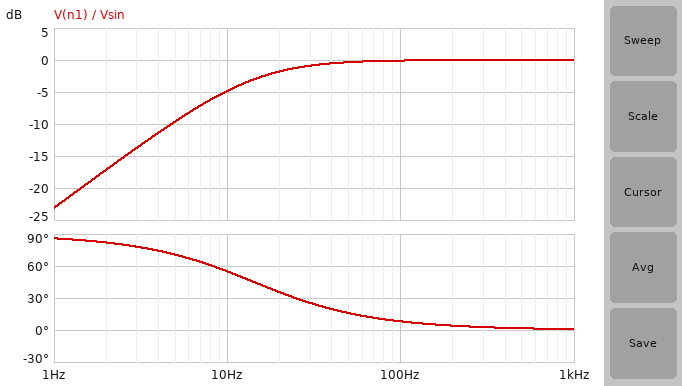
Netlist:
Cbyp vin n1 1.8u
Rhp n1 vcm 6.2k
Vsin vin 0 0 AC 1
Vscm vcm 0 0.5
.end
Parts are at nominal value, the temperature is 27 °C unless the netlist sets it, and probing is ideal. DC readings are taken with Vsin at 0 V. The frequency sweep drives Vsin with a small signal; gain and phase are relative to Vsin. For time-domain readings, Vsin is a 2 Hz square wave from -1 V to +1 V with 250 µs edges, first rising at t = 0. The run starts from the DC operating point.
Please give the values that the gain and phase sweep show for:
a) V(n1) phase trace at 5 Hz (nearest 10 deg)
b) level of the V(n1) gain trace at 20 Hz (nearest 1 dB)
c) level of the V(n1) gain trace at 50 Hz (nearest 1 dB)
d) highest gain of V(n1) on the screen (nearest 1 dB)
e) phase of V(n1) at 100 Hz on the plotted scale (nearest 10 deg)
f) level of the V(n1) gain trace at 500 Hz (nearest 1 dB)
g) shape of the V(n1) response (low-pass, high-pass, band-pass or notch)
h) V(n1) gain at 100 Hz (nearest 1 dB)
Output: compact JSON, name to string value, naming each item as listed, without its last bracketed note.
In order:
{"V(n1) phase trace at 5 Hz": "70 deg", "level of the V(n1) gain trace at 20 Hz": "-2 dB", "level of the V(n1) gain trace at 50 Hz": "0 dB", "highest gain of V(n1) on the screen": "0 dB", "phase of V(n1) at 100 Hz on the plotted scale": "10 deg", "level of the V(n1) gain trace at 500 Hz": "0 dB", "shape of the V(n1) response": "high-pass", "V(n1) gain at 100 Hz": "0 dB"}
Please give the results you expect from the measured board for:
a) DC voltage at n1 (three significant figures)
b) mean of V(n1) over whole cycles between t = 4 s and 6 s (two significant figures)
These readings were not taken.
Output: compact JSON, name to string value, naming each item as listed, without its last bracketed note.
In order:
{"DC voltage at n1": "500 mV", "mean of V(n1) over whole cycles between t = 4 s and 6 s": "500 mV"}
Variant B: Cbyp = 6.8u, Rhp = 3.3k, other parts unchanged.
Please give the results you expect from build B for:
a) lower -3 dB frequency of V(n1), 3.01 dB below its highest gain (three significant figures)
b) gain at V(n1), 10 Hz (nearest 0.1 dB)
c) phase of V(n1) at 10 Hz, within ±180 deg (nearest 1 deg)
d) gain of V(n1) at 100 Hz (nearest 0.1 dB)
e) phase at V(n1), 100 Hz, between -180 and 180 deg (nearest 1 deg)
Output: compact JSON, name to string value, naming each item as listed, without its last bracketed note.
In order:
{"lower -3 dB frequency of V(n1), 3.01 dB below its highest gain": "7.09 Hz", "gain at V(n1), 10 Hz": "-1.8 dB", "phase of V(n1) at 10 Hz, within ±180 deg": "35 deg", "gain of V(n1) at 100 Hz": "0 dB", "phase at V(n1), 100 Hz, between -180 and 180 deg": "4 deg"}
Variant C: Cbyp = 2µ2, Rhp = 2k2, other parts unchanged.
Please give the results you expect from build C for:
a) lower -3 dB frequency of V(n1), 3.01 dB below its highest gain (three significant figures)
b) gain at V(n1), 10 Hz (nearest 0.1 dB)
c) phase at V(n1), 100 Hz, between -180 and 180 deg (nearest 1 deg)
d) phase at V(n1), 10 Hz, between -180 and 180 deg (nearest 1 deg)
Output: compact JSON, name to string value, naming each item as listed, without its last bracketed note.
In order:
{"lower -3 dB frequency of V(n1), 3.01 dB below its highest gain": "32.9 Hz", "gain at V(n1), 10 Hz": "-10.7 dB", "phase at V(n1), 100 Hz, between -180 and 180 deg": "18 deg", "phase at V(n1), 10 Hz, between -180 and 180 deg": "73 deg"}
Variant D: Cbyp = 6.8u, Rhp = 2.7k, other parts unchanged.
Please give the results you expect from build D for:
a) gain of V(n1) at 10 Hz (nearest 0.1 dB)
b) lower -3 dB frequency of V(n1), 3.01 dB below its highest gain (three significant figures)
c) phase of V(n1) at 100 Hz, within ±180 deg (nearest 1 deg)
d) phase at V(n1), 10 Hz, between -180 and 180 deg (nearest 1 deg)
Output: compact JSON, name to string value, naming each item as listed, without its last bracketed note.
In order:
{"gain of V(n1) at 10 Hz": "-2.4 dB", "lower -3 dB frequency of V(n1), 3.01 dB below its highest gain": "8.67 Hz", "phase of V(n1) at 100 Hz, within ±180 deg": "5 deg", "phase at V(n1), 10 Hz, between -180 and 180 deg": "41 deg"}
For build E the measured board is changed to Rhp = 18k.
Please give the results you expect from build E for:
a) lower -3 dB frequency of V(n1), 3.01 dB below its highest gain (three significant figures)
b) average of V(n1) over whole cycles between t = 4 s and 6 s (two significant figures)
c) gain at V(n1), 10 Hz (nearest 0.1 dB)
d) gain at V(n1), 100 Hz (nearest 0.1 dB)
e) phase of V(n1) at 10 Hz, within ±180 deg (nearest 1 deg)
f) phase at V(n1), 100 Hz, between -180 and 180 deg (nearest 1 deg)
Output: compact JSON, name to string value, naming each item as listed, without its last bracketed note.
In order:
{"lower -3 dB frequency of V(n1), 3.01 dB below its highest gain": "4.91 Hz", "average of V(n1) over whole cycles between t = 4 s and 6 s": "500 mV", "gain at V(n1), 10 Hz": "-0.9 dB", "gain at V(n1), 100 Hz": "0 dB", "phase of V(n1) at 10 Hz, within ±180 deg": "26 deg", "phase at V(n1), 100 Hz, between -180 and 180 deg": "3 deg"}
